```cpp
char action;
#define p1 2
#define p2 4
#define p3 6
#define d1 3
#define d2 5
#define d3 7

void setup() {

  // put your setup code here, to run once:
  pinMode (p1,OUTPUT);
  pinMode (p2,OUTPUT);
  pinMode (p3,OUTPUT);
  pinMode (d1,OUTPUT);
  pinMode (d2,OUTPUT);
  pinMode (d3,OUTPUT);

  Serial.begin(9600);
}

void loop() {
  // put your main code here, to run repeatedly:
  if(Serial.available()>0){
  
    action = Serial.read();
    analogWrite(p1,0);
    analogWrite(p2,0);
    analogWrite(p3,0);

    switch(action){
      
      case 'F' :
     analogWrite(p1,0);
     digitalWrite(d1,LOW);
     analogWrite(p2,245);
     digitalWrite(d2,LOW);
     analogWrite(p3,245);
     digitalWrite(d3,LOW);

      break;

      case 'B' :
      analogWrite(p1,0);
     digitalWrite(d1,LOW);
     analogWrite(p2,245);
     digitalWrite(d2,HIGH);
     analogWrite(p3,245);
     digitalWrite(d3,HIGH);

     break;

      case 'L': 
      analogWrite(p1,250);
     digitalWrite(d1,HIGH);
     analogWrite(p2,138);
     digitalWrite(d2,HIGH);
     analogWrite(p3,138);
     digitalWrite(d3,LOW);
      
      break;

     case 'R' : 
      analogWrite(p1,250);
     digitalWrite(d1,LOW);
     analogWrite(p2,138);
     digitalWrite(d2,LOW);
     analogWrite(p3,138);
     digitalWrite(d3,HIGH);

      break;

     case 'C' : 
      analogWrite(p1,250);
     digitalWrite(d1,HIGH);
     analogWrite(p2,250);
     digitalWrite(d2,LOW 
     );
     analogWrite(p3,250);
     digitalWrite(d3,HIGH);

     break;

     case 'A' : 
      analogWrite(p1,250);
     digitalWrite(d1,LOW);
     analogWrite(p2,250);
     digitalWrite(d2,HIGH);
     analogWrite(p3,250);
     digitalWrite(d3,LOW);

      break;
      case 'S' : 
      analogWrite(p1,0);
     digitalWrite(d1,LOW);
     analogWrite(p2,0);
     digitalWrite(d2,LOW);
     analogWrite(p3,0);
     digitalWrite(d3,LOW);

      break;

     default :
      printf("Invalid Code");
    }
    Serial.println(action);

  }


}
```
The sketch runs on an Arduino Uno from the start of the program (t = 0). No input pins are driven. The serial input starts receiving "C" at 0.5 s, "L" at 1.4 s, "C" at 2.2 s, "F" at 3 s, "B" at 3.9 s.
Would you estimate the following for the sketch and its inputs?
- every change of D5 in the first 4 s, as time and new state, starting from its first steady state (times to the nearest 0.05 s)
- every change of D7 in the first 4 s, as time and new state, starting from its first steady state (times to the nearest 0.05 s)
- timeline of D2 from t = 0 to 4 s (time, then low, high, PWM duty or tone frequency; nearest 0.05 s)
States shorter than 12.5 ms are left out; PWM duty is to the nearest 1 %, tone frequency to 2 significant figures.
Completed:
0 s low; 1.4 s high; 2.2 s low; 3.9 s high
0 s low; 0.5 s high; 1.4 s low; 2.2 s high; 3 s low; 3.9 s high
0 s low; 0.5 s high; 3 s low
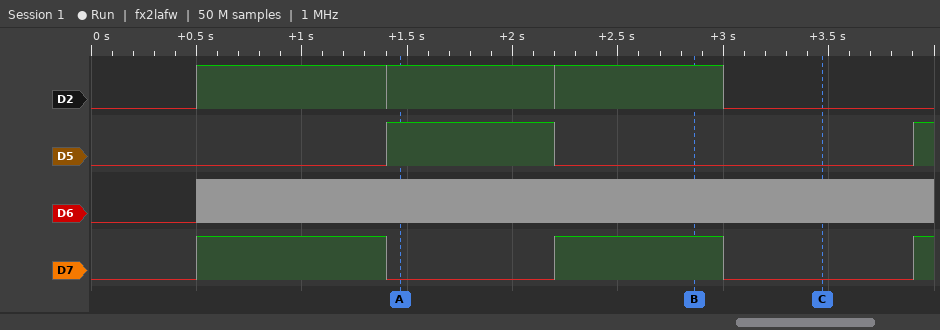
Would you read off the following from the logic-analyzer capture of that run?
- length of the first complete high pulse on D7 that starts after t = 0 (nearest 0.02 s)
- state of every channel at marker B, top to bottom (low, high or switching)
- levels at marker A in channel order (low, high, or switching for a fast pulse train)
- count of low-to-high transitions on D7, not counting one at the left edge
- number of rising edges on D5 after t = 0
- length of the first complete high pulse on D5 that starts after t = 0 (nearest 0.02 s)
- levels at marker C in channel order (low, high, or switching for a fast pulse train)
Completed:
0.90 s
D2 high, D5 low, D6 switching, D7 high
D2 high, D5 high, D6 switching, D7 low
3
2
0.80 s
D2 low, D5 low, D6 switching, D7 low
